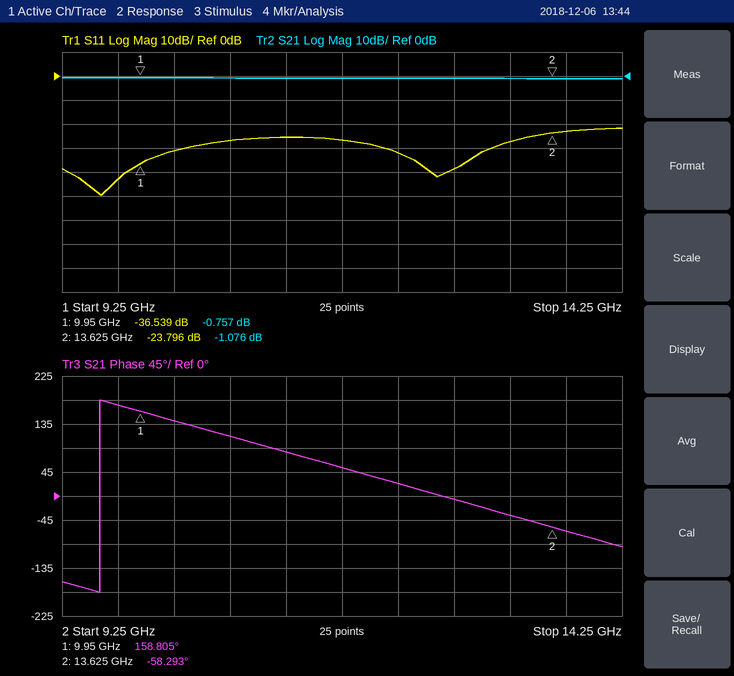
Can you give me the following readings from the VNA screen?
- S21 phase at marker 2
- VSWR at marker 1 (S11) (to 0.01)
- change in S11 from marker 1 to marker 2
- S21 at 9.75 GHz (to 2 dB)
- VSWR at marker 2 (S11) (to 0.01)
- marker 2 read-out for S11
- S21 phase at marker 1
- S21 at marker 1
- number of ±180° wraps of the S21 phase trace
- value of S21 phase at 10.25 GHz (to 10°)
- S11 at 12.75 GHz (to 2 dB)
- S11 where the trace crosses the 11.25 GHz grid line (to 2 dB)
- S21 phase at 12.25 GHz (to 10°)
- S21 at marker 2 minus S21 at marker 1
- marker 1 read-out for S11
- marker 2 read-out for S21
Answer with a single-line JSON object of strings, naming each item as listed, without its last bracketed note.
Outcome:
{"S21 phase at marker 2": "-58.293°", "VSWR at marker 1 (S11)": "1.03", "change in S11 from marker 1 to marker 2": "12.743 dB", "S21 at 9.75 GHz": "0 dB", "VSWR at marker 2 (S11)": "1.14", "marker 2 read-out for S11": "-23.796 dB", "S21 phase at marker 1": "158.805°", "S21 at marker 1": "-0.757 dB", "number of ±180° wraps of the S21 phase trace": "1", "value of S21 phase at 10.25 GHz": "140°", "S11 at 12.75 GHz": "-38 dB", "S11 where the trace crosses the 11.25 GHz grid line": "-26 dB", "S21 phase at 12.25 GHz": "20°", "S21 at marker 2 minus S21 at marker 1": "-0.319 dB", "marker 1 read-out for S11": "-36.539 dB", "marker 2 read-out for S21": "-1.076 dB"}
